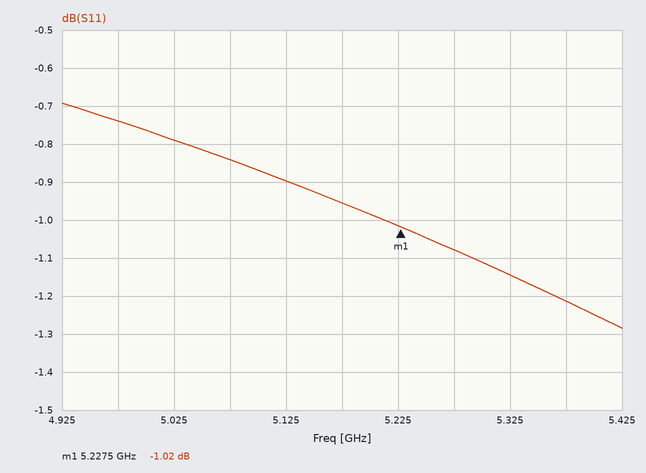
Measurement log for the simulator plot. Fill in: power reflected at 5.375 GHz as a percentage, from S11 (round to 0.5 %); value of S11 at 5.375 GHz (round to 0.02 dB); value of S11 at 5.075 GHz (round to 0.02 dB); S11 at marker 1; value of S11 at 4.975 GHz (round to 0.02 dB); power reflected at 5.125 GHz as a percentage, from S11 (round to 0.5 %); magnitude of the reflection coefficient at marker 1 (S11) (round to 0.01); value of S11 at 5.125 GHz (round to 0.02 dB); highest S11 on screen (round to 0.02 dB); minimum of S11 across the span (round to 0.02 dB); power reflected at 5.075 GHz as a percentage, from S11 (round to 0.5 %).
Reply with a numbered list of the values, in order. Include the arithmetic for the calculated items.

1. 10^(-1.22/10) ≈ 75.5 %
2. -1.22 dB
3. -0.84 dB
4. -1.02 dB
5. -0.74 dB
6. 10^(-0.9/10) ≈ 81.3 %, so 81.5 % to the nearest 0.5 %
7. 10^(-1.02/20) ≈ 0.89
8. -0.90 dB
9. -0.70 dB
10. -1.28 dB
11. 10^(-0.84/10) ≈ 82.4 %, so 82.5 % to the nearest 0.5 %
